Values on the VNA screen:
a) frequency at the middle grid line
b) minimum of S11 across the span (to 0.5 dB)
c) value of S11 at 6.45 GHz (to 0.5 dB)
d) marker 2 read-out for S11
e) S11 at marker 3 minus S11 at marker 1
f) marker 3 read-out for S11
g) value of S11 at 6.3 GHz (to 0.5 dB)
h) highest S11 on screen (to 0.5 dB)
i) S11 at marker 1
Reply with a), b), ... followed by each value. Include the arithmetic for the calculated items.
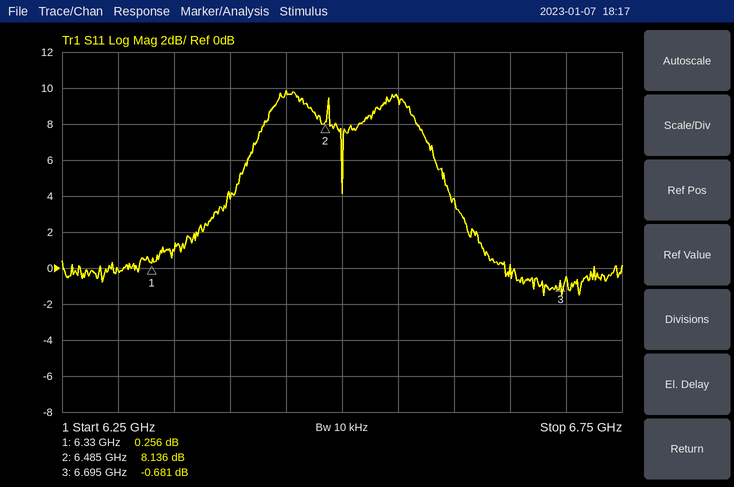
a) 6.5 GHz
b) -1.5 dB
c) 10.0 dB
d) 8.136 dB
e) -0.681 − (0.256) = -0.937 dB
f) -0.681 dB
g) 0.0 dB
h) 10.0 dB
i) 0.256 dB
